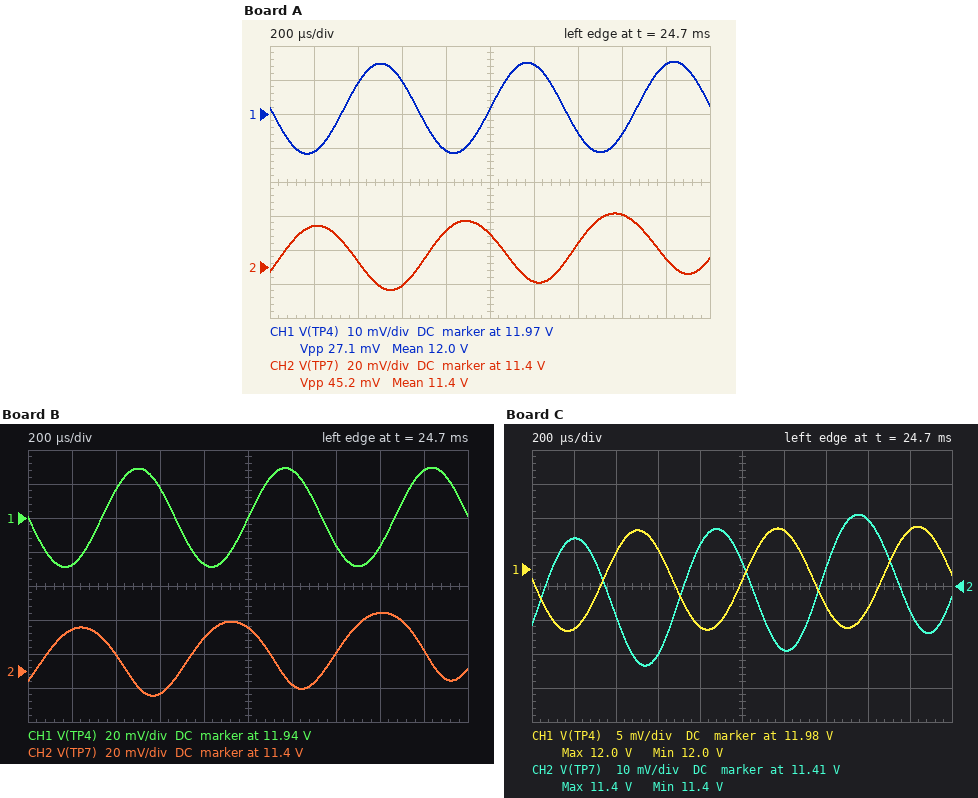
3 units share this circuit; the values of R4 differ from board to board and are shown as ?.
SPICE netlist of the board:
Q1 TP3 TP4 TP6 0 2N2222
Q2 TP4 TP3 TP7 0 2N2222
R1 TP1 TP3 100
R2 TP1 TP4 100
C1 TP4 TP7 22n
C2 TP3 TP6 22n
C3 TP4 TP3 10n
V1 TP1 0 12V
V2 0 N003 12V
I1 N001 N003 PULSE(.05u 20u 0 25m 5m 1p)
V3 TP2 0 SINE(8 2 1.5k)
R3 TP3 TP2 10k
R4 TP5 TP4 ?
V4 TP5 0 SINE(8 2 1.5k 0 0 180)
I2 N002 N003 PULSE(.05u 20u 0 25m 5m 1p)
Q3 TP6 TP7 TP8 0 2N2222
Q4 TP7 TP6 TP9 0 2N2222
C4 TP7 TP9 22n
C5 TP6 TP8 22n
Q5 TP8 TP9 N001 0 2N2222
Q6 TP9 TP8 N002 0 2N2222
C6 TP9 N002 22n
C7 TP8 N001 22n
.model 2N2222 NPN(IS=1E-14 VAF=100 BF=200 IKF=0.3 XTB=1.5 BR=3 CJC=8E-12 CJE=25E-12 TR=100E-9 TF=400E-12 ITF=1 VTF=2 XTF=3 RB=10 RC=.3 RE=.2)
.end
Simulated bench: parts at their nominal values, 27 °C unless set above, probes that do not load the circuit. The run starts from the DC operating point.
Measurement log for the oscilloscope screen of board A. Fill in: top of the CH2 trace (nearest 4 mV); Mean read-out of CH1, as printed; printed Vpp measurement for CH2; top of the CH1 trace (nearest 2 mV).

11.432 V
12.0 V
45.2 mV
11.986 V
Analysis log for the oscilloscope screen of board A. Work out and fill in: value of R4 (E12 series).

15 kΩ
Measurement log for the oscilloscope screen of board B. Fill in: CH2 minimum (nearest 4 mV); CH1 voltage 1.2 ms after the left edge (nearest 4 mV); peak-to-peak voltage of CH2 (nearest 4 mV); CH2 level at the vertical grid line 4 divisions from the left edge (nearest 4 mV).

11.384 V
11.968 V
48 mV
11.420 V
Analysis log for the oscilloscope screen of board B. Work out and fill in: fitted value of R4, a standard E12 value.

6.8 kΩ
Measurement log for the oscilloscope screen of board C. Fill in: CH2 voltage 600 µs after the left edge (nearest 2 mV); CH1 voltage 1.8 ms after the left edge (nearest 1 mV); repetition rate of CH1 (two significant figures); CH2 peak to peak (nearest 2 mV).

11.390 V
11.991 V
1.5 kHz
44 mV
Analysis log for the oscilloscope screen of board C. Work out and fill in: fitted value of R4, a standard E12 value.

27 kΩ
